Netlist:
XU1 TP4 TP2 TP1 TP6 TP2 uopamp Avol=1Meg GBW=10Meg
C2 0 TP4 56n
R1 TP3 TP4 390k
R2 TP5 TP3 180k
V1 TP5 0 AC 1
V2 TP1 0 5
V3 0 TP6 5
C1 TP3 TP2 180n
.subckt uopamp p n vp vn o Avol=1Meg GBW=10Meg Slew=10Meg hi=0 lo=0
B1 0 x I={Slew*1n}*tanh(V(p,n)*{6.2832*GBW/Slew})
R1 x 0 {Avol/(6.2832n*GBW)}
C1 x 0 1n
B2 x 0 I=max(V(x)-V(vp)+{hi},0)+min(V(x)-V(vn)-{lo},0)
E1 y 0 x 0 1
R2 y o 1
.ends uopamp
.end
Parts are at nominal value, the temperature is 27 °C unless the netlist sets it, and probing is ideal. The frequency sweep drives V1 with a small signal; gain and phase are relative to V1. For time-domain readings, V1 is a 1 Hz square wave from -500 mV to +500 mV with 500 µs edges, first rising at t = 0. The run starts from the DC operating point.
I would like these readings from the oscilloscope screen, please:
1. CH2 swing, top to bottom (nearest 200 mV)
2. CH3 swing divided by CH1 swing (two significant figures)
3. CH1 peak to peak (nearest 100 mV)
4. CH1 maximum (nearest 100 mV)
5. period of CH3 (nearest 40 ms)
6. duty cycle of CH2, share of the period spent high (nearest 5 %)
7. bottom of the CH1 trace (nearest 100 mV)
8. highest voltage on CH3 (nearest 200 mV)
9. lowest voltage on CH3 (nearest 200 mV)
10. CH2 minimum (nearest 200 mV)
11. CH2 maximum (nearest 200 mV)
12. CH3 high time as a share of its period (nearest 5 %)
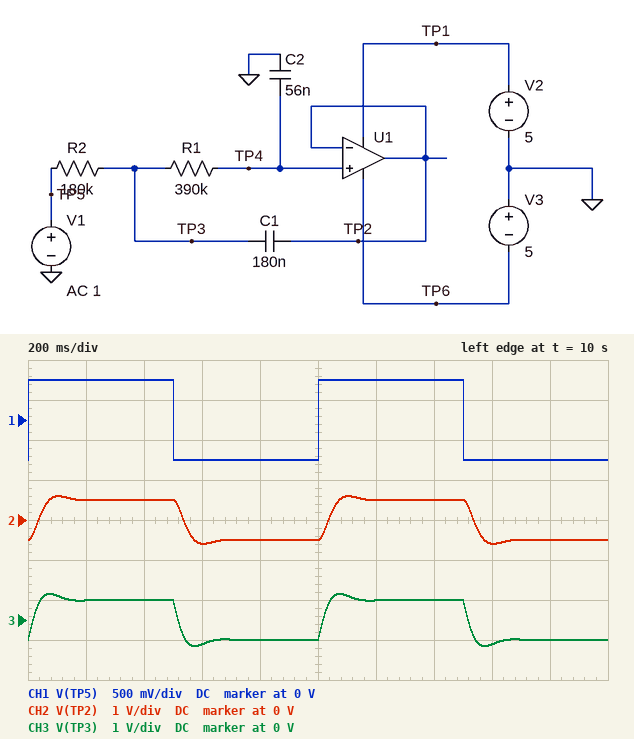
1.2 V
1.3
1.0 V
500 mV
1.00 s
50 %
-500 mV
600 mV
-600 mV
-600 mV
600 mV
50 %
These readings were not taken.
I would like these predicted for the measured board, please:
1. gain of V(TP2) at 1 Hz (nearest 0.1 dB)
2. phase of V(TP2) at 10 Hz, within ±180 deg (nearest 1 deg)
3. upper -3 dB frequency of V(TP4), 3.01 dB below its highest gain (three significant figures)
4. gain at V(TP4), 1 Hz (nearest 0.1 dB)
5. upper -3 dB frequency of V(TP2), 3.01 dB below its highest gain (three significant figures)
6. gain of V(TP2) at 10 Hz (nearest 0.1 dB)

0.1 dB
-132 deg
6.66 Hz
0.1 dB
6.66 Hz
-8.6 dB
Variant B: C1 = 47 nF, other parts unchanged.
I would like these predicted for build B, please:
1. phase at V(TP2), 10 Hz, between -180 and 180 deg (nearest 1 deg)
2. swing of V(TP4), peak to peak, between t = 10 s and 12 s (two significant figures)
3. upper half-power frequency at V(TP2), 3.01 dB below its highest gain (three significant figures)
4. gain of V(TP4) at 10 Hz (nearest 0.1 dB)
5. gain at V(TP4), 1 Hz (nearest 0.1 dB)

-82 deg
1.0 V
6.02 Hz
-6.1 dB
-0.1 dB
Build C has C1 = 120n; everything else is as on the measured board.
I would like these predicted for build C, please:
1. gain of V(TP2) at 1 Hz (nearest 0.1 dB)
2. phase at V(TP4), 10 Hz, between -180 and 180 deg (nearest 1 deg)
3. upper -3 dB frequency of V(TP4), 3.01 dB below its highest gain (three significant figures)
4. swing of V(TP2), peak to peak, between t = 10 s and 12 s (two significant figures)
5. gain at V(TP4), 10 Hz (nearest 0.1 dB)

0 dB
-113 deg
7.04 Hz
1.1 V
-6.8 dB
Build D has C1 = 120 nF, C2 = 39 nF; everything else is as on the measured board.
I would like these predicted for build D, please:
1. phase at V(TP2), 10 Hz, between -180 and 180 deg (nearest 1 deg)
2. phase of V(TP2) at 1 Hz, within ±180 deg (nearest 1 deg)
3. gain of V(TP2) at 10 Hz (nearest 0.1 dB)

-102 deg
-8 deg
-3.1 dB
